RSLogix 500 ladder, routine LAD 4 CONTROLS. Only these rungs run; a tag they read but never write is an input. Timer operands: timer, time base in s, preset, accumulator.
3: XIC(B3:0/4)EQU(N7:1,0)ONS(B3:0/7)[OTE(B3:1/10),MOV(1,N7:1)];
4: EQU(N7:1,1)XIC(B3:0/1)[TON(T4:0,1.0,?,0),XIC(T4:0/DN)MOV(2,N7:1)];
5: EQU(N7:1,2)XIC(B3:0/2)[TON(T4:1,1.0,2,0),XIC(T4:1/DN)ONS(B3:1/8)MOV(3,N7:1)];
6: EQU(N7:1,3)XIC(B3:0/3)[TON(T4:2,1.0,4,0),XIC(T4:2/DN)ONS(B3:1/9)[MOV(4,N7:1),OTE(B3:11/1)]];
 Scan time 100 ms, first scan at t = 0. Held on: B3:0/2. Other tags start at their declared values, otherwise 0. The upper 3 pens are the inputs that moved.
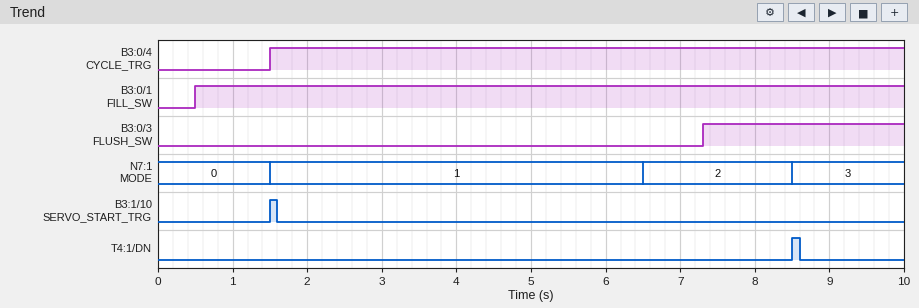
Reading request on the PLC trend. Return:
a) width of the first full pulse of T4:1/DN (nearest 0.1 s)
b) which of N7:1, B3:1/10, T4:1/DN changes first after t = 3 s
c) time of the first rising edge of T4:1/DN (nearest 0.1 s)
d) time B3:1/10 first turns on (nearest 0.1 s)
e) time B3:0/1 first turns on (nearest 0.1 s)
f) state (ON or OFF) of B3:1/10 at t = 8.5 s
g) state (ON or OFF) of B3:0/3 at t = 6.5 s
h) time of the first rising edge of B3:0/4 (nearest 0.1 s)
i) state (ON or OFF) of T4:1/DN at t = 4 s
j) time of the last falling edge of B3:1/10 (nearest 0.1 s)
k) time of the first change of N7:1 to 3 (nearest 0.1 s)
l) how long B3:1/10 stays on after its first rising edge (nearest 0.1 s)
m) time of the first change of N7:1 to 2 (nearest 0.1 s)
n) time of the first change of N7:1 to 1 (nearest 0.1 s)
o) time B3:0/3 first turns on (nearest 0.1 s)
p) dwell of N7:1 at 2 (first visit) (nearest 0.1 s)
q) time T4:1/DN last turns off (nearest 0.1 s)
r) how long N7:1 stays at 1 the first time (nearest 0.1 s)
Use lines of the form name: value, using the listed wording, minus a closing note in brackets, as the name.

width of the first full pulse of T4:1/DN: 0.1 s
which of N7:1, B3:1/10, T4:1/DN changes first after t = 3 s: N7:1
time of the first rising edge of T4:1/DN: 8.5 s
time B3:1/10 first turns on: 1.5 s
time B3:0/1 first turns on: 0.5 s
state (ON or OFF) of B3:1/10 at t = 8.5 s: OFF
state (ON or OFF) of B3:0/3 at t = 6.5 s: OFF
time of the first rising edge of B3:0/4: 1.5 s
state (ON or OFF) of T4:1/DN at t = 4 s: OFF
time of the last falling edge of B3:1/10: 1.6 s
time of the first change of N7:1 to 3: 8.5 s
how long B3:1/10 stays on after its first rising edge: 0.1 s
time of the first change of N7:1 to 2: 6.5 s
time of the first change of N7:1 to 1: 1.5 s
time B3:0/3 first turns on: 7.3 s
dwell of N7:1 at 2 (first visit): 2.0 s
time T4:1/DN last turns off: 8.6 s
how long N7:1 stays at 1 the first time: 5.0 s
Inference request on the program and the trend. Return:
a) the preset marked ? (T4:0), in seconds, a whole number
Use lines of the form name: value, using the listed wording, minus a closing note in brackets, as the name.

the preset marked ? (T4:0), in seconds, a whole number: 5 s
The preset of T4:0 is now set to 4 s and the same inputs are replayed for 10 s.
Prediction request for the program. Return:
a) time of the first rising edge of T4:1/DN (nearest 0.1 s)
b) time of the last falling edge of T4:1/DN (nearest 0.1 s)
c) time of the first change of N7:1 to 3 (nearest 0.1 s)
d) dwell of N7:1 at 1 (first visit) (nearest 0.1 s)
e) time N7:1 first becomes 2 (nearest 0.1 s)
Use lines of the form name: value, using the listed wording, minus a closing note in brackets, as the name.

time of the first rising edge of T4:1/DN: 7.5 s
time of the last falling edge of T4:1/DN: 7.6 s
time of the first change of N7:1 to 3: 7.5 s
dwell of N7:1 at 1 (first visit): 4.0 s
time N7:1 first becomes 2: 5.5 s
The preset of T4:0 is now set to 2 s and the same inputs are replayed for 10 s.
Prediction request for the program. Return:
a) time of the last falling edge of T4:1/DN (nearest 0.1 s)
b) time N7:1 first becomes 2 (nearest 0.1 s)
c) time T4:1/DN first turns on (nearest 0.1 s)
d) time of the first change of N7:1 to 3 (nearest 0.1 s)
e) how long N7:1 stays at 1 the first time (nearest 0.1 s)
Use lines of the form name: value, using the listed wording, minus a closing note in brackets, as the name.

time of the last falling edge of T4:1/DN: 5.6 s
time N7:1 first becomes 2: 3.5 s
time T4:1/DN first turns on: 5.5 s
time of the first change of N7:1 to 3: 5.5 s
how long N7:1 stays at 1 the first time: 2.0 s
